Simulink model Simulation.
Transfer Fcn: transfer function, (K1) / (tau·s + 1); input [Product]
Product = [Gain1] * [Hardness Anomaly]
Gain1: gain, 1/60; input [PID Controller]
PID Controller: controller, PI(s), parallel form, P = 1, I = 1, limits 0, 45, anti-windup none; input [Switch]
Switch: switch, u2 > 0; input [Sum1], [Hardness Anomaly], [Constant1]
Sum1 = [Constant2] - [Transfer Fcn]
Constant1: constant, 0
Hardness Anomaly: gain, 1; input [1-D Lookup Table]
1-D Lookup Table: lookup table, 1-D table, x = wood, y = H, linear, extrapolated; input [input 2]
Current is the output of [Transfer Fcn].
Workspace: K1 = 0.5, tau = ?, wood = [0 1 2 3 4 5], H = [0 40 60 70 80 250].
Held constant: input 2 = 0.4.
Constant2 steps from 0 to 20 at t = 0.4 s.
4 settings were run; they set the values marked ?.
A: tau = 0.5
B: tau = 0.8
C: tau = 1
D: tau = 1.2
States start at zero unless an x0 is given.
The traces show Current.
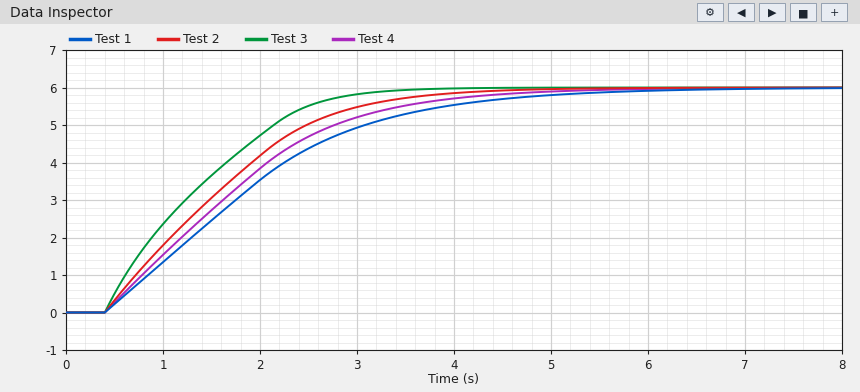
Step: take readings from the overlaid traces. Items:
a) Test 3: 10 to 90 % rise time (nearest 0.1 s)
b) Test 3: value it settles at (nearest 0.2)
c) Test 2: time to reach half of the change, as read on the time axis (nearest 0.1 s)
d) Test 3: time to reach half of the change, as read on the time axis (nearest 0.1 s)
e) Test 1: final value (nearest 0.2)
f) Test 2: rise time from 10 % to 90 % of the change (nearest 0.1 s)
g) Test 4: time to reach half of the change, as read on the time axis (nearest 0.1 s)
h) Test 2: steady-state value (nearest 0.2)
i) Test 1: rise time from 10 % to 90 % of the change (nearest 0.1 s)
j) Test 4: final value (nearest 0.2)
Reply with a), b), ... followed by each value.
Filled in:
a) 1.9 s
b) 6.0
c) 1.5 s
d) 1.2 s
e) 6.0
f) 2.3 s
g) 1.6 s
h) 6.0
i) 3.0 s
j) 6.0
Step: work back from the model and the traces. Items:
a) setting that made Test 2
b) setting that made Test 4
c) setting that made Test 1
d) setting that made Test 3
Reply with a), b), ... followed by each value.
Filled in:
a) B
b) C
c) D
d) A
